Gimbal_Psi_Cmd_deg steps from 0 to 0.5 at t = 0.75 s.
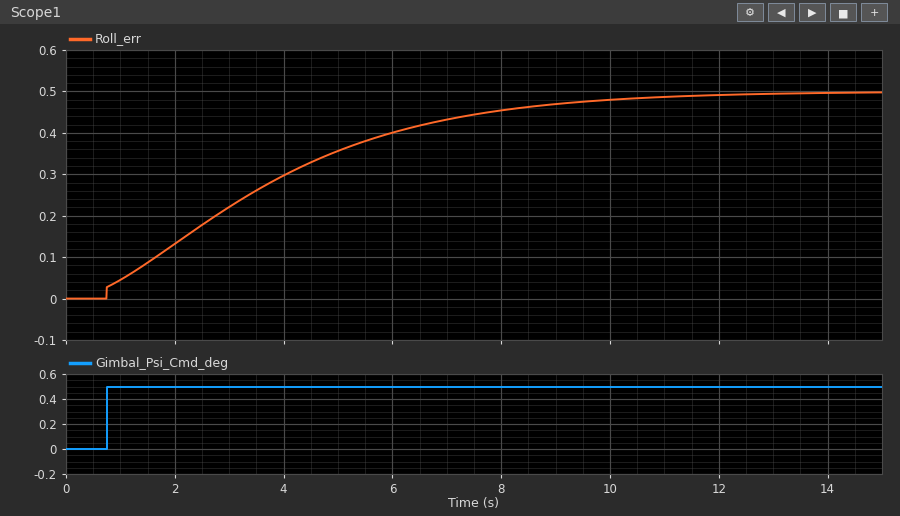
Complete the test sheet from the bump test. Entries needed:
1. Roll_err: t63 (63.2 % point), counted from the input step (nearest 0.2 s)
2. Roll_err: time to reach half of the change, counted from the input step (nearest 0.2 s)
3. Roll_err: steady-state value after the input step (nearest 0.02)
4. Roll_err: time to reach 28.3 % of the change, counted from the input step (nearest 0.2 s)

3.6 s
2.6 s
0.50
1.4 s
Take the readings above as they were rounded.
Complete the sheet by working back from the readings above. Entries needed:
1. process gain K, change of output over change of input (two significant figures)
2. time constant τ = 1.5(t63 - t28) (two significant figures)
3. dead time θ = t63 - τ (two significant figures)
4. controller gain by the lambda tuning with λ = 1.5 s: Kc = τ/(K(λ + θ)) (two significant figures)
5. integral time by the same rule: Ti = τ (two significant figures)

1.0
3.3 s
0.30 s
1.8
3.3 s
